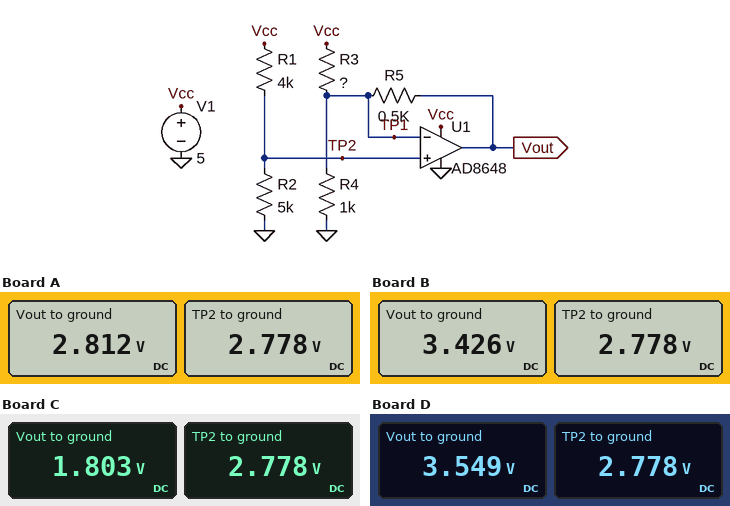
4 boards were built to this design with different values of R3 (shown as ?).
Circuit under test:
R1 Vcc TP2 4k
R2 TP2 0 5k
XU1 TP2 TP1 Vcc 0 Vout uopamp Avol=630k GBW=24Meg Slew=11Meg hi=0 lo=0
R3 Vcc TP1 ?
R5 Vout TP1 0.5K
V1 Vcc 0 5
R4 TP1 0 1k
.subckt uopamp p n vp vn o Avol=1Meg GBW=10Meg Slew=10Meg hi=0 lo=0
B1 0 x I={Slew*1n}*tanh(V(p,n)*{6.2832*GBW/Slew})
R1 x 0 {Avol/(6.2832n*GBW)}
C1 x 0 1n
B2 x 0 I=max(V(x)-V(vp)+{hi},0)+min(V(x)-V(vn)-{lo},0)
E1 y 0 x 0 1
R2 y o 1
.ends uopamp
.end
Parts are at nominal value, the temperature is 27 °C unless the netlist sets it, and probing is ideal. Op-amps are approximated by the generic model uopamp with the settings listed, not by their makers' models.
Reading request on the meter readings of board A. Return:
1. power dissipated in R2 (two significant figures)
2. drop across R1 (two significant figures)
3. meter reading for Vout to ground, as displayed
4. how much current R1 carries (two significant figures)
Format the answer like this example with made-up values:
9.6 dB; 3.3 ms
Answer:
1.5 mW; 2.2 V; 2.812 V; 560 µA
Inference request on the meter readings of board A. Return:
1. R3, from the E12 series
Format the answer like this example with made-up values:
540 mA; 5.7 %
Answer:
820 Ω
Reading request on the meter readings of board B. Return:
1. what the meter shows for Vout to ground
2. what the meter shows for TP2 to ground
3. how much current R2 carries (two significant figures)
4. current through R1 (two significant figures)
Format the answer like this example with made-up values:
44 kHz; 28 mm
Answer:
3.426 V; 2.778 V; 560 µA; 560 µA
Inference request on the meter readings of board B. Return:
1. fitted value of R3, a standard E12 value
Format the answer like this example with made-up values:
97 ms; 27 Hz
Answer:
1.5 kΩ
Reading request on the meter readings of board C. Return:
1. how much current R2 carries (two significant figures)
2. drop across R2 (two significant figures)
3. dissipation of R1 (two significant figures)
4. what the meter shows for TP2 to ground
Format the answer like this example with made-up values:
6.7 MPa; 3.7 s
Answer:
560 µA; 2.8 V; 1.2 mW; 2.778 V
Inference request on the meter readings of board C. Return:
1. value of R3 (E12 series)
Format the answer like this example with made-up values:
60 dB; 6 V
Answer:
470 Ω
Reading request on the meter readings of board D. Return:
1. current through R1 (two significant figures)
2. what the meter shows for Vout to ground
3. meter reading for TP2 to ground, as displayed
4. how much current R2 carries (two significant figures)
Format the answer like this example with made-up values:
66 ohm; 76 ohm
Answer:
560 µA; 3.549 V; 2.778 V; 560 µA
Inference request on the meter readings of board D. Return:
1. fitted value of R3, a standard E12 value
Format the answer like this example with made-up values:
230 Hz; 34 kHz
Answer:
1.8 kΩ
